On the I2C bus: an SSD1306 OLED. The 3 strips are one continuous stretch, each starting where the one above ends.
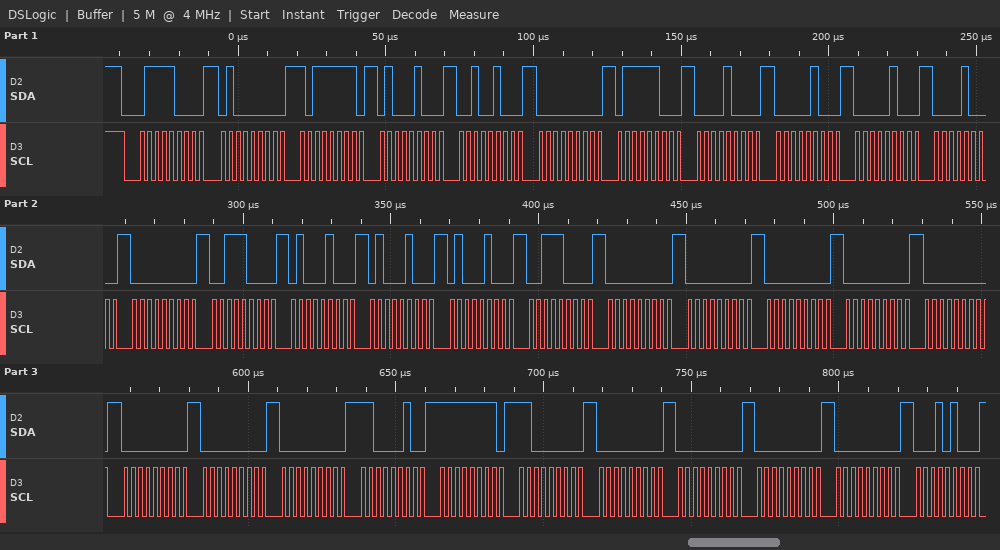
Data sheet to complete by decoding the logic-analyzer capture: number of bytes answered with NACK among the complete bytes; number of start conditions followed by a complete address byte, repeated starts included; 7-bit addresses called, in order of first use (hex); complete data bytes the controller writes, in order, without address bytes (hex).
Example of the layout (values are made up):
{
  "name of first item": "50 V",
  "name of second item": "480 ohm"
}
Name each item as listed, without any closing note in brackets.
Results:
{
  "number of bytes answered with NACK among the complete bytes": "0",
  "number of start conditions followed by a complete address byte, repeated starts included": "1",
  "7-bit addresses called, in order of first use": "0x3C",
  "complete data bytes the controller writes, in order, without address bytes": "40 BF 44 24 00 7C 08 04 04 08 00 38 44 44 44 38 00 00 00 00 00 00 00 00 C2 FF C0 00 00 00 00 14"
}
